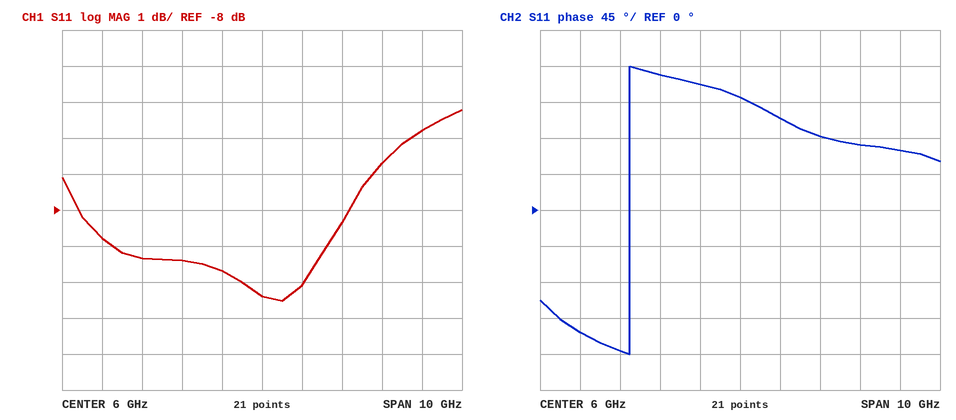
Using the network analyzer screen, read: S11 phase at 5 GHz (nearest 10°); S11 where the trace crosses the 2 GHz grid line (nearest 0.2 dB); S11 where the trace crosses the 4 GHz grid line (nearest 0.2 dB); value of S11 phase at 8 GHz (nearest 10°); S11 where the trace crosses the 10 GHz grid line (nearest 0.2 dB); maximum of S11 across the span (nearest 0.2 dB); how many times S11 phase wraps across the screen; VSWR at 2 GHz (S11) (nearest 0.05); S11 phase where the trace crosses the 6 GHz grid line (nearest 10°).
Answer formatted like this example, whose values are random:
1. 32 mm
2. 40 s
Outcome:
1. 160°
2. -8.8 dB
3. -9.4 dB
4. 90°
5. -5.8 dB
6. -5.2 dB
7. 1
8. 2.15
9. 140°
